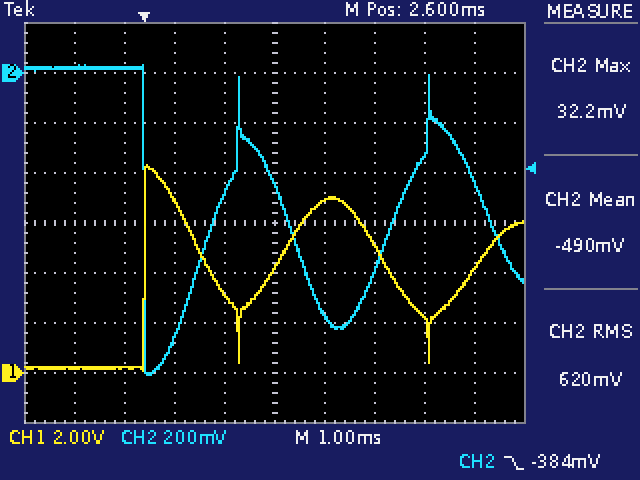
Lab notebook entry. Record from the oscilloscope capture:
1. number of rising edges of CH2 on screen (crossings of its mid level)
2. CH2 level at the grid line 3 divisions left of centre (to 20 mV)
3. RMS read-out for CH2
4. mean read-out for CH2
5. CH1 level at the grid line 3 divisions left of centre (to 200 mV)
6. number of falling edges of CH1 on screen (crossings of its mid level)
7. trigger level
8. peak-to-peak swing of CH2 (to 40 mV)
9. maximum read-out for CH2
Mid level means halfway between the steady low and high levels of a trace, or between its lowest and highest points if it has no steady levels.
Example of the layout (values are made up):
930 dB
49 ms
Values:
2
20 mV
620 mV
-490 mV
200 mV
2
-384 mV
1.24 V
32.2 mV
